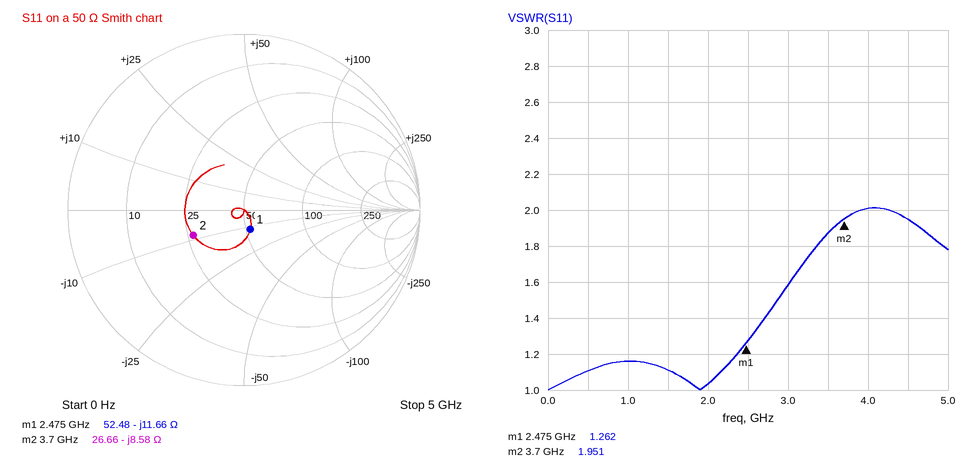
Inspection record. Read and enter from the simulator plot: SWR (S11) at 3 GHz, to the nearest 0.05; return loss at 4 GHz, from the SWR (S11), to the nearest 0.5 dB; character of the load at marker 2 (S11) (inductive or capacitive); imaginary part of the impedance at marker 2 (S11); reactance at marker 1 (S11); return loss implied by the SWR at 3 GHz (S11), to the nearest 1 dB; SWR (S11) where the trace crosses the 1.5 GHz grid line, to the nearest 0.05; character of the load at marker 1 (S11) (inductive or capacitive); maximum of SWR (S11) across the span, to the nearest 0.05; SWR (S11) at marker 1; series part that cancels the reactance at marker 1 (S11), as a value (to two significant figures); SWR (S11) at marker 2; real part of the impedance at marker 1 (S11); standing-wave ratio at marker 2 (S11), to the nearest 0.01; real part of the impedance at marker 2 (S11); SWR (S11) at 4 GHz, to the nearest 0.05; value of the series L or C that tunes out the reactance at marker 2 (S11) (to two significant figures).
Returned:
1.60
9.5 dB
capacitive
-8.58 Ω
-11.66 Ω
13 dB
1.10
capacitive
2.00
1.262
750 pH
1.951
52.48 Ω
1.95
26.66 Ω
2.00
370 pH
